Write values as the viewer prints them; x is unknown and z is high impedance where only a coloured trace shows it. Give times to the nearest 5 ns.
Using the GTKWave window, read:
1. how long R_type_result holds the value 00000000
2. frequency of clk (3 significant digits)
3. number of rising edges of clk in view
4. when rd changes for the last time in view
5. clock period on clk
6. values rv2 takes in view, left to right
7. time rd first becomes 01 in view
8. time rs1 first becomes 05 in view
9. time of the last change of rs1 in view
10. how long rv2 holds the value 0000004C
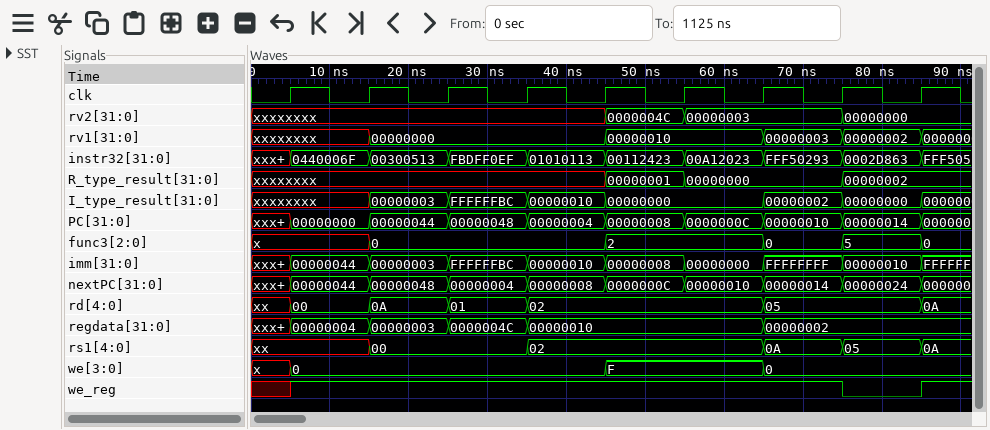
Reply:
20 ns
100 MHz
9
85 ns
10 ns
xxxxxxxx, 0000004C, 00000003, 00000000
25 ns
75 ns
85 ns
10 ns
